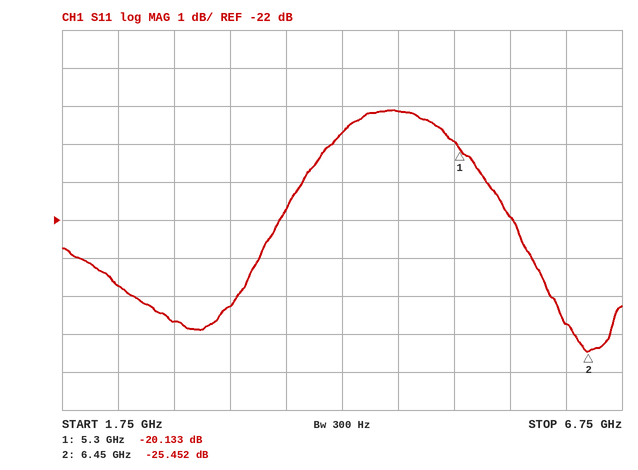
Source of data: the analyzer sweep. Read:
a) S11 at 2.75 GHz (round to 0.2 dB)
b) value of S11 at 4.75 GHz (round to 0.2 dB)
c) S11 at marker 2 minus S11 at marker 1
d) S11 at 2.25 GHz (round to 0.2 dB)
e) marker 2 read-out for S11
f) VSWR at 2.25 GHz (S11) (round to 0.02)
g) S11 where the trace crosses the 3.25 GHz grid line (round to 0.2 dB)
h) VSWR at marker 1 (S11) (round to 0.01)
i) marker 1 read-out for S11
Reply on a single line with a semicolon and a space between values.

-24.6 dB; -19.2 dB; -5.319 dB; -23.8 dB; -25.452 dB; 1.14; -24.2 dB; 1.22; -20.133 dB
